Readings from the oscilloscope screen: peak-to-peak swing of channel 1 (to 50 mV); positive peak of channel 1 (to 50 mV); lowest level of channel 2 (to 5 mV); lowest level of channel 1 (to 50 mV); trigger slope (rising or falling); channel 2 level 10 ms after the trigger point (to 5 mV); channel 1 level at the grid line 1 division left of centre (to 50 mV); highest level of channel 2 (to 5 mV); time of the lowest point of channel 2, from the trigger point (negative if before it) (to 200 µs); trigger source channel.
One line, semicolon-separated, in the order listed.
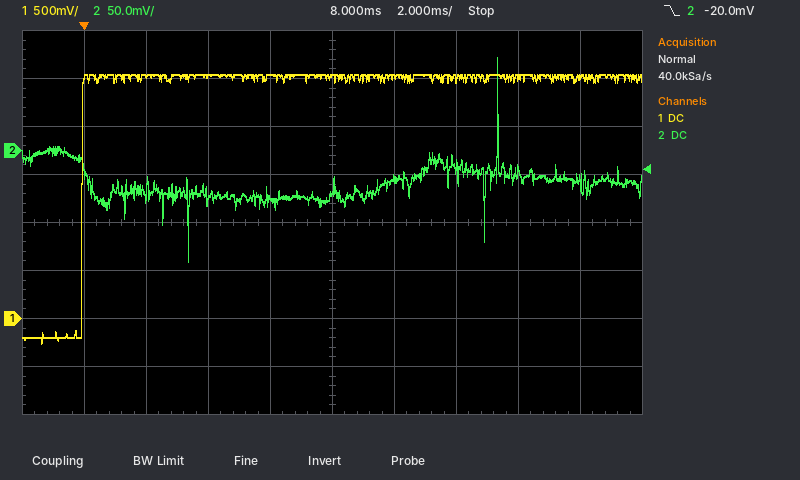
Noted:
2.80 V; 2.55 V; -115 mV; -250 mV; falling; -30 mV; 2.55 V; 95 mV; +3.4 ms; channel 2
